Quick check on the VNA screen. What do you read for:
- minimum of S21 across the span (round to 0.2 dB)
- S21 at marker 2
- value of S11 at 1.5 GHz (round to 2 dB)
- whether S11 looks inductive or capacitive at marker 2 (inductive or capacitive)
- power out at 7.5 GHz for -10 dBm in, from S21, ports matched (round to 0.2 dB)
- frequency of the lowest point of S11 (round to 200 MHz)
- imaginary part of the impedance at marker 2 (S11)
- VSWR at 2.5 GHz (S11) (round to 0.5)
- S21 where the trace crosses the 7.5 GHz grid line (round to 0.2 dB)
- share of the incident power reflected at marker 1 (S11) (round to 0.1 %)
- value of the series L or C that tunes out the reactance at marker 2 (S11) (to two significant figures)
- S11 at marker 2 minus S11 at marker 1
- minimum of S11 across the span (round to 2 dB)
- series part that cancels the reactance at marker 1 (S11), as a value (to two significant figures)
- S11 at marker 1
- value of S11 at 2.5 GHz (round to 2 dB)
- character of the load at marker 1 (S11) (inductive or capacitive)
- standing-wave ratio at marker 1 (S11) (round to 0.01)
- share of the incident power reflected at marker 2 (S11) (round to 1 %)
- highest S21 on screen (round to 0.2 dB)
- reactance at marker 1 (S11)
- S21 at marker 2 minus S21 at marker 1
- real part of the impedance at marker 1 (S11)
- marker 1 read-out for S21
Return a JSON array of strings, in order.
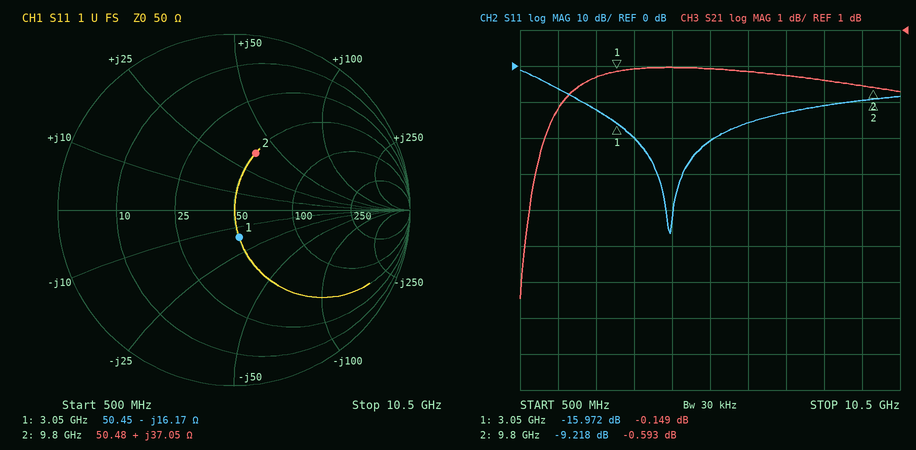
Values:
["-6.4 dB", "-0.593 dB", "-6 dB", "inductive", "-10.2 dBm", "4.4 GHz", "+37.05 Ω", "1.5", "-0.2 dB", "2.5 %", "440 fF", "6.754 dB", "-46 dB", "840 pH", "-15.972 dB", "-12 dB", "capacitive", "1.38", "12 %", "0.0 dB", "-16.17 Ω", "-0.444 dB", "50.45 Ω", "-0.149 dB"]
